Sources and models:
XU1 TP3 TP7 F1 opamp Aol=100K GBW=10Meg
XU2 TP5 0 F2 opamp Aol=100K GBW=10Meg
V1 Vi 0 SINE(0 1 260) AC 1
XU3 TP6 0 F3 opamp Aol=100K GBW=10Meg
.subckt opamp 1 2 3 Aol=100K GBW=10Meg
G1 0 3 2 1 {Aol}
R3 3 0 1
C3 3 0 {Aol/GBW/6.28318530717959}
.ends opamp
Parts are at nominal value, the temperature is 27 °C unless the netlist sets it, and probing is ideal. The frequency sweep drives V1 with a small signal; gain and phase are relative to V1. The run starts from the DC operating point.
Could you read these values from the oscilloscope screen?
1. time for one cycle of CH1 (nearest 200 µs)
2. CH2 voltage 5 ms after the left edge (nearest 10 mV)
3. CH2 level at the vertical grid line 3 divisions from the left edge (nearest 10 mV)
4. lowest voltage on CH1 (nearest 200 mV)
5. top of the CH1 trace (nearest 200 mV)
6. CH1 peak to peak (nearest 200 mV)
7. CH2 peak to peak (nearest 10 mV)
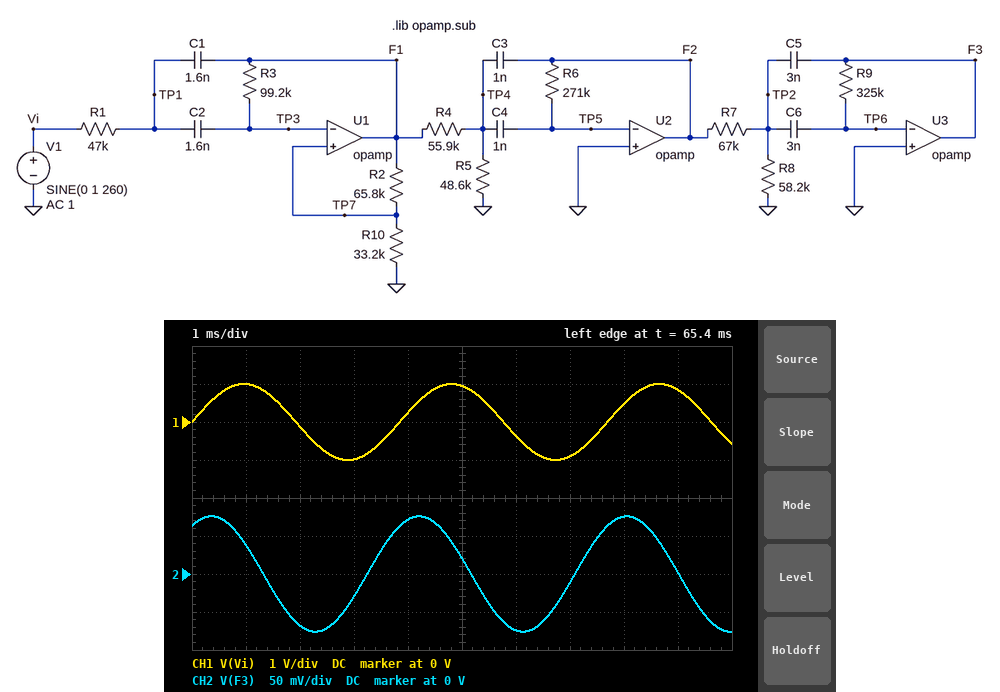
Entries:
3.8 ms
20 mV
-30 mV
-1.0 V
1.0 V
2.0 V
150 mV
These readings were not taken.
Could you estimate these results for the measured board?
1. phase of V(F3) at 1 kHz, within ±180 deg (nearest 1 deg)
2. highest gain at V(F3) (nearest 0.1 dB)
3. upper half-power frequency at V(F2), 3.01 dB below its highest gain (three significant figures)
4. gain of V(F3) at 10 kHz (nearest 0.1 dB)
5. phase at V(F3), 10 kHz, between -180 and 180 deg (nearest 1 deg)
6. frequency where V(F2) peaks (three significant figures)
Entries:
-130 deg
11.6 dB
2.12 kHz
-42.5 dB
-76 deg
1.67 kHz
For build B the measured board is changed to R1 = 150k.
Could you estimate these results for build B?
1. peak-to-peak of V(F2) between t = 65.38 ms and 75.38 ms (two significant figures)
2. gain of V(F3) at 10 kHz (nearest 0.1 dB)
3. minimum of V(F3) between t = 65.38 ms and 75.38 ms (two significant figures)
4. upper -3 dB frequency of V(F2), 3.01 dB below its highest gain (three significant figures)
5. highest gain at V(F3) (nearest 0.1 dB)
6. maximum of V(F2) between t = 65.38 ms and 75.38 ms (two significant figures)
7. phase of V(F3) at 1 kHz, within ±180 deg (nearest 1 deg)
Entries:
150 mV
-52.8 dB
-67 mV
2.32 kHz
-3.6 dB
73 mV
169 deg
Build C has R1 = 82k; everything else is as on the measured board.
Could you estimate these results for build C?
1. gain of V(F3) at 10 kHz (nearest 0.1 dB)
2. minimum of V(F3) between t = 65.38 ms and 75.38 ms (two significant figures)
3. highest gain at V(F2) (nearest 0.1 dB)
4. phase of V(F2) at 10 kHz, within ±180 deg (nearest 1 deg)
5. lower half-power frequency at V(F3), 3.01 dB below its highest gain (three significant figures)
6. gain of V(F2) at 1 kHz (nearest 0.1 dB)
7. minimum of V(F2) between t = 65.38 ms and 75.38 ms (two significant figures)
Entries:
-47.4 dB
-75 mV
7.8 dB
-165 deg
552 Hz
2.2 dB
-82 mV
